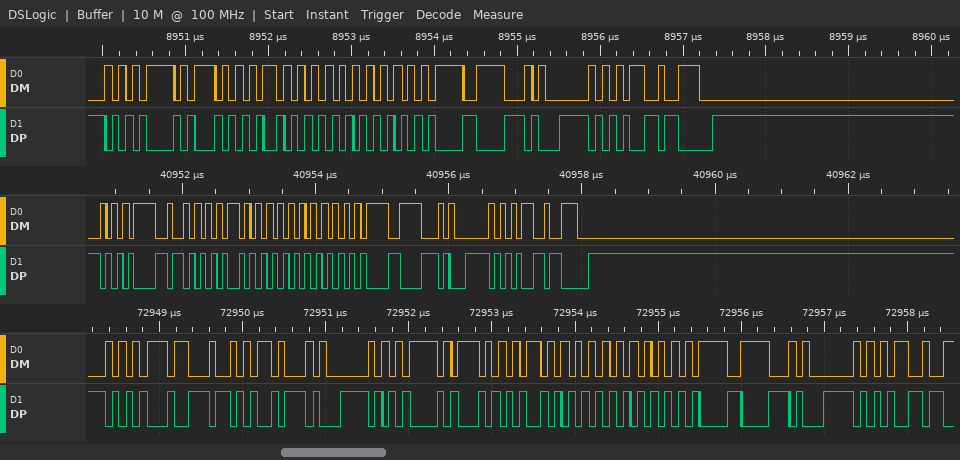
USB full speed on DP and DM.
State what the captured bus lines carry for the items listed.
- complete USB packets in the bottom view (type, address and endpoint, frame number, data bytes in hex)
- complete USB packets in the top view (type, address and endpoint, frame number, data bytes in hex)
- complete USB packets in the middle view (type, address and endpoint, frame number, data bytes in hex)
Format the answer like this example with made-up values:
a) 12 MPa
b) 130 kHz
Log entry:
a) IN ADDR 2 EP 1, DATA0 [ 00 01 00 00 ]
b) DATA0 [ 00 01 00 00 ], ACK
c) DATA1 [ 00 01 00 00 ], ACK
